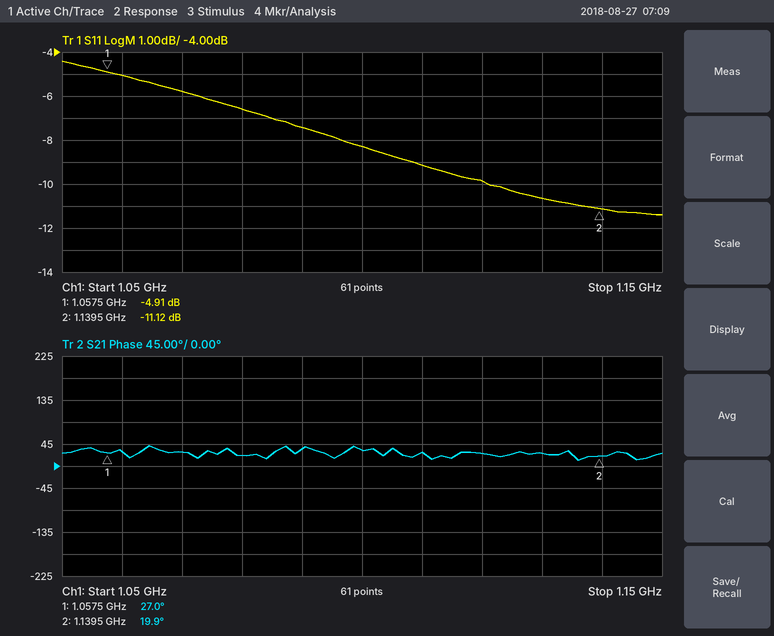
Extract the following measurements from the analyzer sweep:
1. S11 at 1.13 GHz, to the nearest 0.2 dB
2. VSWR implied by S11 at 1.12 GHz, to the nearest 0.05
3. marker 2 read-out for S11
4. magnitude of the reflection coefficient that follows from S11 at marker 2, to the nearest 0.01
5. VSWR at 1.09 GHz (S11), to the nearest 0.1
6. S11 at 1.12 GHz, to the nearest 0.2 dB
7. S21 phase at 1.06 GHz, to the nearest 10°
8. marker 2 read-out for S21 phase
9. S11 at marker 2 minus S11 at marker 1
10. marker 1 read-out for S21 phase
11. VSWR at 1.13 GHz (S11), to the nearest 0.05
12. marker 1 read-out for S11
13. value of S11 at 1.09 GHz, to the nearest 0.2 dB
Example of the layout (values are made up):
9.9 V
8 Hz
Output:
-10.6 dB
1.95
-11.12 dB
0.28
2.5
-9.8 dB
30°
19.9°
-6.21 dB
27.0°
1.85
-4.91 dB
-7.4 dB
